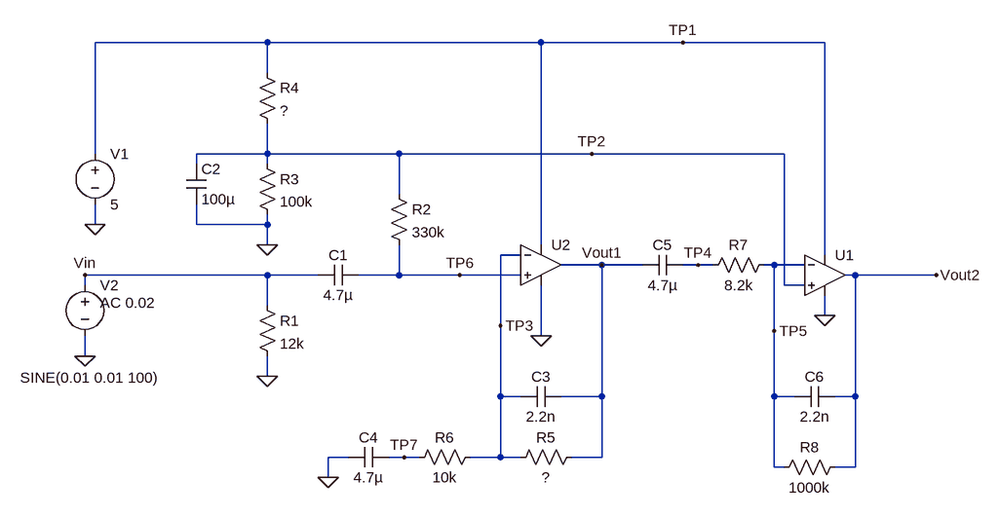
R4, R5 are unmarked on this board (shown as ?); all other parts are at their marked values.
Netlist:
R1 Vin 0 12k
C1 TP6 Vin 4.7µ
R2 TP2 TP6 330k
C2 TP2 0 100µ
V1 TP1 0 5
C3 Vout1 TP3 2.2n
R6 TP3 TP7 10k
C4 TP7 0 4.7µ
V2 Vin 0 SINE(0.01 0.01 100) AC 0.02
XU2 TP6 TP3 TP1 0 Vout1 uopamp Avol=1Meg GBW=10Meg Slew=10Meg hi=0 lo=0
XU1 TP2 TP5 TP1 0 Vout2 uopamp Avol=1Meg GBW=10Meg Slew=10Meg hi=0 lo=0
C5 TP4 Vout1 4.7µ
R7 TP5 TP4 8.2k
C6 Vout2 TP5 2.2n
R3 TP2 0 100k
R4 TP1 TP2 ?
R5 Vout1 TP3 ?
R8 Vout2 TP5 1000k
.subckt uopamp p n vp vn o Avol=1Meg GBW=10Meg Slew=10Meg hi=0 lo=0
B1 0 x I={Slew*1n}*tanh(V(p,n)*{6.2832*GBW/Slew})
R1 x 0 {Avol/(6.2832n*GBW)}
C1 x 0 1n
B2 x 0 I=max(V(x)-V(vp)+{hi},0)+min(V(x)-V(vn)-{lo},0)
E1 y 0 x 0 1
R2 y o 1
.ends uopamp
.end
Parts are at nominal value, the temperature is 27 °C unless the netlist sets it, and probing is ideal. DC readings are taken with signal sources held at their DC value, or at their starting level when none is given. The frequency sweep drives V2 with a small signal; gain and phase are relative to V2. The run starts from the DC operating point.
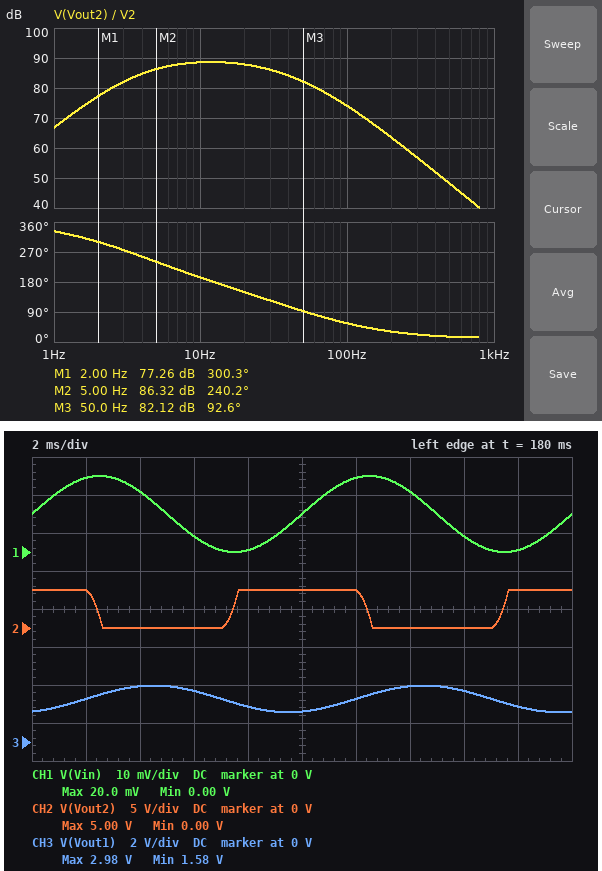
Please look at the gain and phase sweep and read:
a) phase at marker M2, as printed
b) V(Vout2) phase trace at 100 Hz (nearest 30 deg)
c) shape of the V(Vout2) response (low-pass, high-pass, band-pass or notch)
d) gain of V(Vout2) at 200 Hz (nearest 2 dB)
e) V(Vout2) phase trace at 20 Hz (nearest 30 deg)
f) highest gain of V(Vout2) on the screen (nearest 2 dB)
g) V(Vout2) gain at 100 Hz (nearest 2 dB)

240.2 deg
60 deg
band-pass
64 dB
150 deg
88 dB
74 dB
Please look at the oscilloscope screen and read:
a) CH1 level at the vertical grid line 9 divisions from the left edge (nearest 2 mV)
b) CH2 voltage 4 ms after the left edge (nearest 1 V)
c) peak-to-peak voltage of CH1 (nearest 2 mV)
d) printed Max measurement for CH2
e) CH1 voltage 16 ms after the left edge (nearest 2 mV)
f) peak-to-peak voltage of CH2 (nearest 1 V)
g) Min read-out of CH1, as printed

0 V
0 V
20 mV
5.00 V
4 mV
5 V
0.00 V
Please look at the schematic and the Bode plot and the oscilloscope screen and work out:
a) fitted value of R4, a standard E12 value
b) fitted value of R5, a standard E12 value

120 kΩ
2.7 MΩ
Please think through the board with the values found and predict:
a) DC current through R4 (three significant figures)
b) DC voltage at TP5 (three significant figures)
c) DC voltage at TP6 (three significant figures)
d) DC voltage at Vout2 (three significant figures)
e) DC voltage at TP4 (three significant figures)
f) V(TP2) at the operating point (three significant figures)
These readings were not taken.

22.7 µA
2.27 V
2.27 V
2.27 V
2.27 V
2.27 V
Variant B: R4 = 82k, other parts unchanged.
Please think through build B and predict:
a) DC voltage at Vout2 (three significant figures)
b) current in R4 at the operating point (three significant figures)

2.75 V
27.5 µA
